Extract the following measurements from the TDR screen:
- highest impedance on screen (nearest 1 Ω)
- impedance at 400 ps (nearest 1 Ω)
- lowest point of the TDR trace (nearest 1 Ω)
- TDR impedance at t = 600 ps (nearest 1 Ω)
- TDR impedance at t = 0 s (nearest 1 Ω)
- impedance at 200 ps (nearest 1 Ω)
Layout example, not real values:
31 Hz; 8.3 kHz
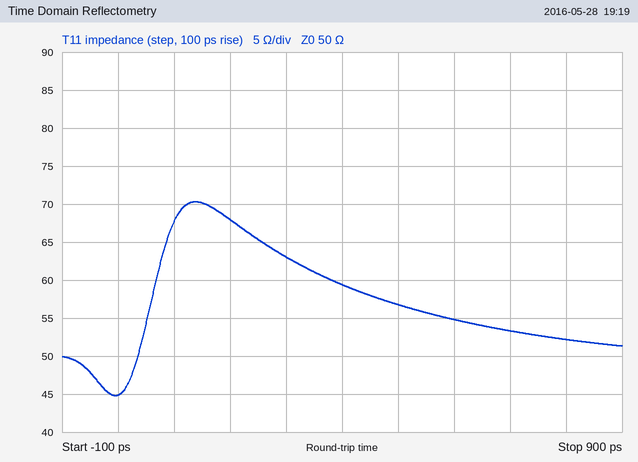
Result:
70 Ω; 59 Ω; 45 Ω; 55 Ω; 45 Ω; 68 Ω
